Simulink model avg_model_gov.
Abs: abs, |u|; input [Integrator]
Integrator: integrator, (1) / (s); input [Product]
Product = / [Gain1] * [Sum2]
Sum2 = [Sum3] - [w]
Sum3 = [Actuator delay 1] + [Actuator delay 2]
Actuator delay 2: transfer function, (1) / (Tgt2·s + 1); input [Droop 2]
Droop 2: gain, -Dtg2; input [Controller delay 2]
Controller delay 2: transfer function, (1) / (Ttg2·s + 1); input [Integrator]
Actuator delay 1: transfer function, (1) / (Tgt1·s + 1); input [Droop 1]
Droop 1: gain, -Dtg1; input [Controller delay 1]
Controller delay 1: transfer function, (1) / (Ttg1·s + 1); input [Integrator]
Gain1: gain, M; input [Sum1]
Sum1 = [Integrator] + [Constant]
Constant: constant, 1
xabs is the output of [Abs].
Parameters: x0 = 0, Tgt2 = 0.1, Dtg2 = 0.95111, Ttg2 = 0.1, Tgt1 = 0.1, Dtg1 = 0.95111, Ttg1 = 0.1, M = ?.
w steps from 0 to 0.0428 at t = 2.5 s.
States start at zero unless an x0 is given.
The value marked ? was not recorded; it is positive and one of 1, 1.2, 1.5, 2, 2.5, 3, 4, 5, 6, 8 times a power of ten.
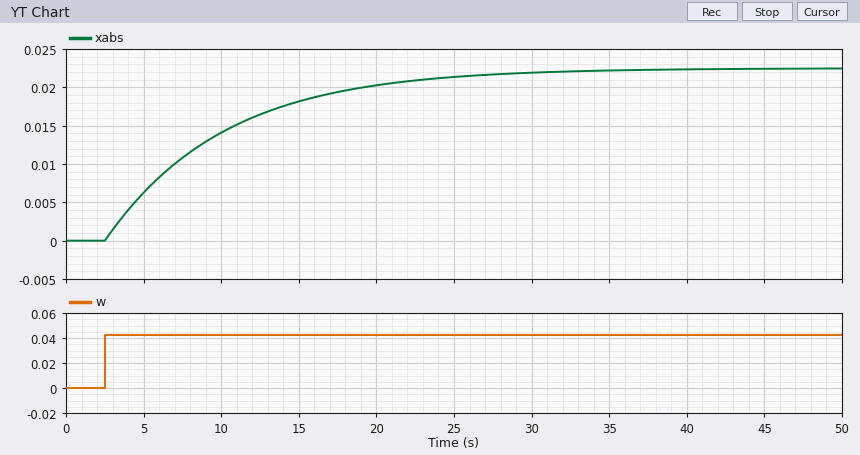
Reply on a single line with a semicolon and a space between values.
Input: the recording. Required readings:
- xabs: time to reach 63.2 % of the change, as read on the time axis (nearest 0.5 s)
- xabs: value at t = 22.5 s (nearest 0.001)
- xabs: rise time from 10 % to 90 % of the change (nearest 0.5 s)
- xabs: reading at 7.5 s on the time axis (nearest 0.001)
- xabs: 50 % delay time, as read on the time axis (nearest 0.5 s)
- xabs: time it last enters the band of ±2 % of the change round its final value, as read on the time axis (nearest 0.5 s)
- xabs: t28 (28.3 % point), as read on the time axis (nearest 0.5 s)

10.0 s; 0.021; 16.5 s; 0.011; 8.0 s; 32.0 s; 5.0 s
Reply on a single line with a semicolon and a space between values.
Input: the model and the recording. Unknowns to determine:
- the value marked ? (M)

15
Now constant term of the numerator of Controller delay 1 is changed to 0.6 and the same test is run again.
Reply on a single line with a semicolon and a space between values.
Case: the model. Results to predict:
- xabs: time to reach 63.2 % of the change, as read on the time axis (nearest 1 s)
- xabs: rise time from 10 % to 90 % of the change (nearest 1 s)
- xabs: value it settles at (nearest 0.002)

12 s; 21 s; 0.028
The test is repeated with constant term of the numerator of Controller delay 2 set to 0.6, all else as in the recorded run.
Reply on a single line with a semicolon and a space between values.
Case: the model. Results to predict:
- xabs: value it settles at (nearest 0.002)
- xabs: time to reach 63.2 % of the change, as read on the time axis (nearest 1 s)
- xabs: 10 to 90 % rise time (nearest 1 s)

0.028; 12 s; 21 s
